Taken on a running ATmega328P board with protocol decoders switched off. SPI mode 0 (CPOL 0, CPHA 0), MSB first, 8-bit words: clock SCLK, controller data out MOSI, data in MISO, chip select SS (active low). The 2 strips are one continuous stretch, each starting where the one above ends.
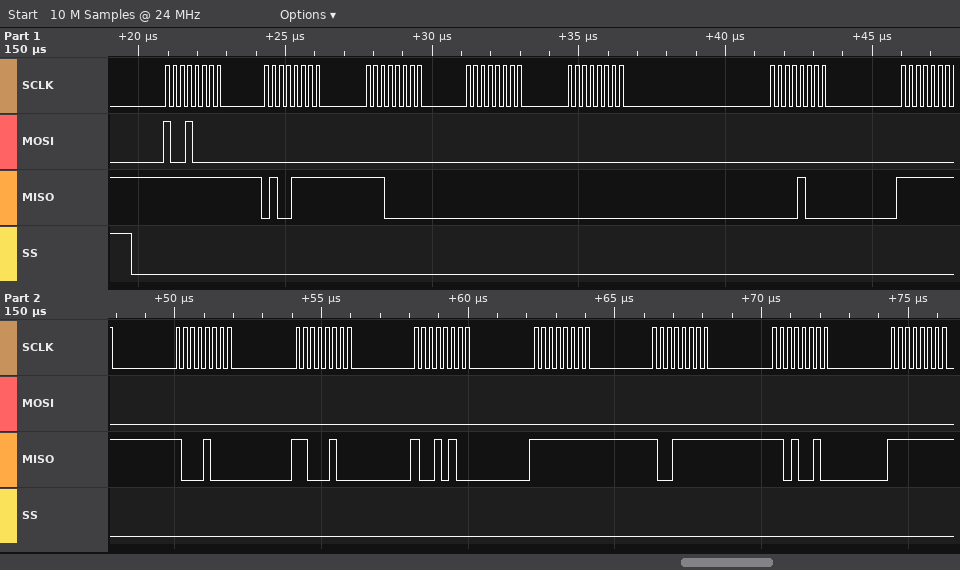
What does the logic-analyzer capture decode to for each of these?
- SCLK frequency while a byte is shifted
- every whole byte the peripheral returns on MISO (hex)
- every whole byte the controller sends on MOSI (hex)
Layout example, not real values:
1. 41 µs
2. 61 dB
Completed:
1. 4 MHz
2. FF 4F E0 00 00 08 FF 88 C4 94 FF 9F D2 FF
3. 90 00 00 00 00 00 00 00 00 00 00 00 00 00
